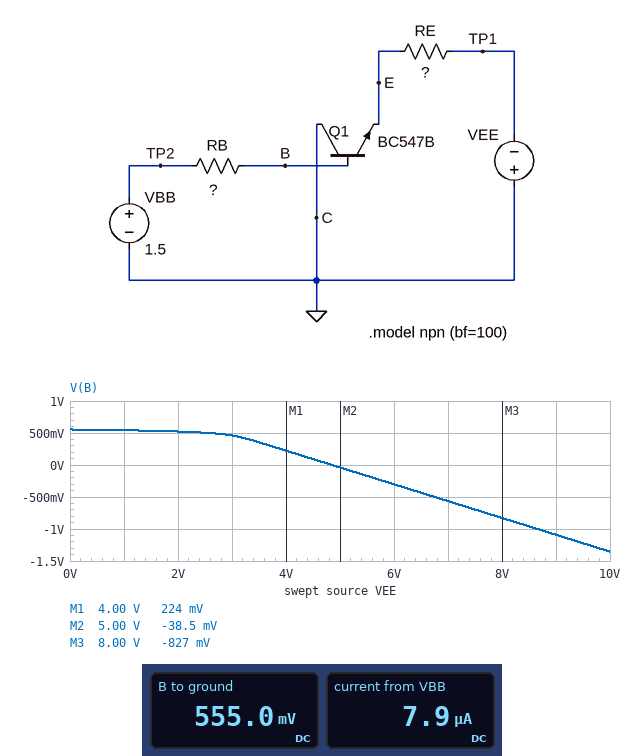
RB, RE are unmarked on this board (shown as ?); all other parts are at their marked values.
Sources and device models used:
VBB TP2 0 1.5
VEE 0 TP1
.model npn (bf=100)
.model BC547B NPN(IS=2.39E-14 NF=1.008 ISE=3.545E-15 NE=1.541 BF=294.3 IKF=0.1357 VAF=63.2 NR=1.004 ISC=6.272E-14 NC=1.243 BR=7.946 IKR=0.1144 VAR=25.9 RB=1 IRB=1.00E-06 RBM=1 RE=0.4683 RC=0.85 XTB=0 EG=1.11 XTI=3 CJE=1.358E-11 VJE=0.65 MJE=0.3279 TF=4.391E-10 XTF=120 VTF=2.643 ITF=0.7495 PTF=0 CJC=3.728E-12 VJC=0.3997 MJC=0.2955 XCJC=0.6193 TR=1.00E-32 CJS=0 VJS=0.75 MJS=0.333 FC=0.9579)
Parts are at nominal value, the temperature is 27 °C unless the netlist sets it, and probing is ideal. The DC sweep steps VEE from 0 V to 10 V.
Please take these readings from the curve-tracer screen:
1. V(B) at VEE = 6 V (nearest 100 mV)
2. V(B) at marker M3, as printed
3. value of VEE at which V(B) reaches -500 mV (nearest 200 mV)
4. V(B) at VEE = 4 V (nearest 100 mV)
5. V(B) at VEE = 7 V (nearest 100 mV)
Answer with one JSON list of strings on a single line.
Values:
["-300 mV", "-827 mV", "6.8 V", "200 mV", "-600 mV"]
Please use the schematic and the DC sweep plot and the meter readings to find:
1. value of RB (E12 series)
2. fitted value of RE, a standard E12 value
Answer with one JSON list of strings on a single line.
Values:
["120 kΩ", "1.2 kΩ"]
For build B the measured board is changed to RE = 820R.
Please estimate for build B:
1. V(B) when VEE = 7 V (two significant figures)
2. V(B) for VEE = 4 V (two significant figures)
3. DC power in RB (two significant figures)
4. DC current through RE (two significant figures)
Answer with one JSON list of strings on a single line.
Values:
["-1.2 V", "-160 mV", "7.4 µW", "1.5 µA"]
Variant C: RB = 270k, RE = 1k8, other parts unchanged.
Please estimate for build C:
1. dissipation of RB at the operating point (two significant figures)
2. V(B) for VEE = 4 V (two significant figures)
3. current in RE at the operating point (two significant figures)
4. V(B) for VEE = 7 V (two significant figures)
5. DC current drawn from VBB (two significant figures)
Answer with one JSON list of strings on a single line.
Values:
["3.5 µW", "-180 mV", "640 nA", "-1.2 V", "3.6 µA"]
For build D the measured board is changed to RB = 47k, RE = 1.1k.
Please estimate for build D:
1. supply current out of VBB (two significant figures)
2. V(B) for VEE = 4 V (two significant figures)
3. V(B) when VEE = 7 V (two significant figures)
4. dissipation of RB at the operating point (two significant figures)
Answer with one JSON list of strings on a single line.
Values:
["20 µA", "550 mV", "430 mV", "18 µW"]
